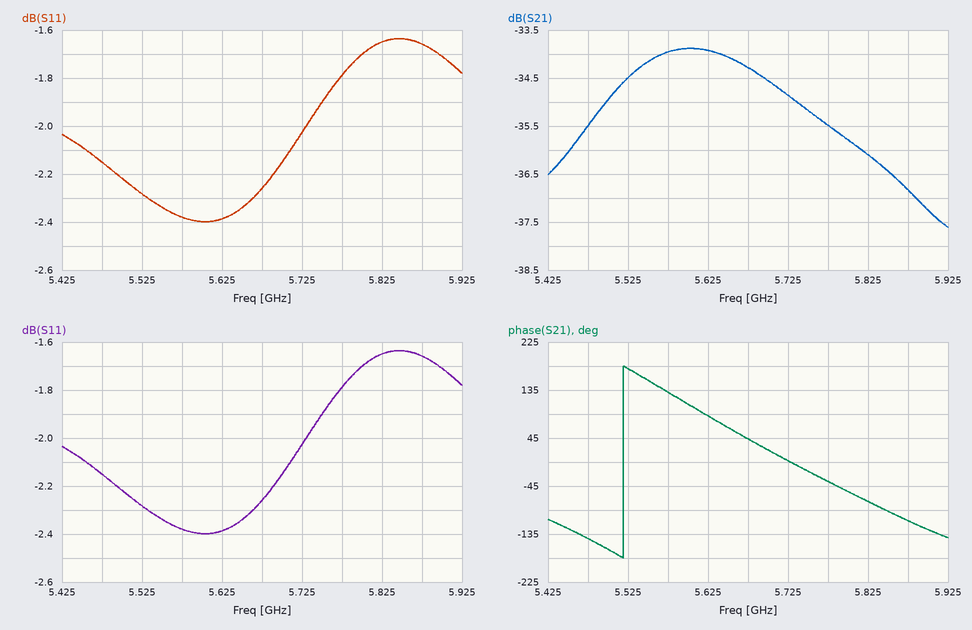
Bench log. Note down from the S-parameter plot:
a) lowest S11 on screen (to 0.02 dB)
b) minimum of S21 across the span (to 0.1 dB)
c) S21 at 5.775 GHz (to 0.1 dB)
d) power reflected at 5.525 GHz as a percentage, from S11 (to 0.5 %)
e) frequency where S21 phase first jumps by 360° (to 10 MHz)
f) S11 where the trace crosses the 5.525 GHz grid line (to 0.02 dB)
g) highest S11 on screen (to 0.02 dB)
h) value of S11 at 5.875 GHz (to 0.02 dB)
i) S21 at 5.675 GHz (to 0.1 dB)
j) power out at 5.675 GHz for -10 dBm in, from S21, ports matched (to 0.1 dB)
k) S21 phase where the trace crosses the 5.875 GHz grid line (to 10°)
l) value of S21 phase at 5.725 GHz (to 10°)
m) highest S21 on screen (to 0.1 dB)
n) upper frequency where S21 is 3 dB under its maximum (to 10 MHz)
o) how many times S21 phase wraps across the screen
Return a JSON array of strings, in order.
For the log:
["-2.40 dB", "-37.6 dB", "-35.5 dB", "59.0 %", "5.52 GHz", "-2.28 dB", "-1.64 dB", "-1.66 dB", "-34.3 dB", "-44.3 dBm", "-110°", "0°", "-33.9 dB", "5.88 GHz", "1"]
